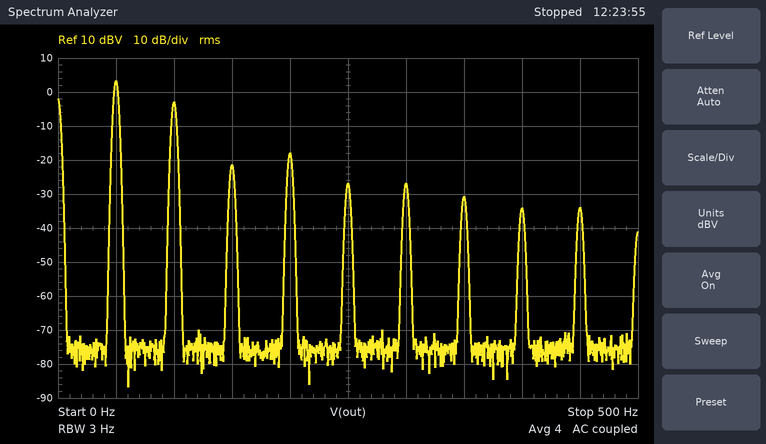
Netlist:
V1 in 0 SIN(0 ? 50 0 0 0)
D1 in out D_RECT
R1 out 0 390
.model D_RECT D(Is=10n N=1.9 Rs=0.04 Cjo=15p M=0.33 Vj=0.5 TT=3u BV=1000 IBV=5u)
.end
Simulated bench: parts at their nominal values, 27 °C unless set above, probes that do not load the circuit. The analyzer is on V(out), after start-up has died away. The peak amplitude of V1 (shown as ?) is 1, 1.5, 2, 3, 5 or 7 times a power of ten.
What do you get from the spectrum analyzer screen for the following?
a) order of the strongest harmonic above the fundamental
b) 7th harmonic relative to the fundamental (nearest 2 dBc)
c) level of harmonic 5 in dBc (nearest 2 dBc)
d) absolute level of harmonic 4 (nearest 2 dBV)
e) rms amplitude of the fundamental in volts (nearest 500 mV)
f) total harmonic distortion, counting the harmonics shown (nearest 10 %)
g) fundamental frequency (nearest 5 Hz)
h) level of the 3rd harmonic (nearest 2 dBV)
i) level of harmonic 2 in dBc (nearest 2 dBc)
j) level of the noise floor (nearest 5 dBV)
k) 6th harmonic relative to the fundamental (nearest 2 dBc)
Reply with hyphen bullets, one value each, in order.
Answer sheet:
- 2
- -34 dBc
- -30 dBc
- -18 dBV
- 1.5 V
- 50 %
- 50 Hz
- -22 dBV
- -6 dBc
- -75 dBV
- -30 dBc
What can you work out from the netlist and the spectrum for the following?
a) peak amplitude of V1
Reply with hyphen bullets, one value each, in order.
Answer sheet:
- 5 V
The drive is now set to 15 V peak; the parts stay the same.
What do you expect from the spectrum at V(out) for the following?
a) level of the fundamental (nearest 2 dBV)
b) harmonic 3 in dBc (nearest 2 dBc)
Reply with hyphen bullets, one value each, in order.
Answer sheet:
- 14 dBV
- -34 dBc
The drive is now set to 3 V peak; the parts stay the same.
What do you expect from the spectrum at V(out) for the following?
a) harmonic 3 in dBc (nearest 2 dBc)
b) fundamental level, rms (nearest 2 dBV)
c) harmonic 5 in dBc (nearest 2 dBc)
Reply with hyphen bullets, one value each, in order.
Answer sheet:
- -20 dBc
- -2 dBV
- -26 dBc
